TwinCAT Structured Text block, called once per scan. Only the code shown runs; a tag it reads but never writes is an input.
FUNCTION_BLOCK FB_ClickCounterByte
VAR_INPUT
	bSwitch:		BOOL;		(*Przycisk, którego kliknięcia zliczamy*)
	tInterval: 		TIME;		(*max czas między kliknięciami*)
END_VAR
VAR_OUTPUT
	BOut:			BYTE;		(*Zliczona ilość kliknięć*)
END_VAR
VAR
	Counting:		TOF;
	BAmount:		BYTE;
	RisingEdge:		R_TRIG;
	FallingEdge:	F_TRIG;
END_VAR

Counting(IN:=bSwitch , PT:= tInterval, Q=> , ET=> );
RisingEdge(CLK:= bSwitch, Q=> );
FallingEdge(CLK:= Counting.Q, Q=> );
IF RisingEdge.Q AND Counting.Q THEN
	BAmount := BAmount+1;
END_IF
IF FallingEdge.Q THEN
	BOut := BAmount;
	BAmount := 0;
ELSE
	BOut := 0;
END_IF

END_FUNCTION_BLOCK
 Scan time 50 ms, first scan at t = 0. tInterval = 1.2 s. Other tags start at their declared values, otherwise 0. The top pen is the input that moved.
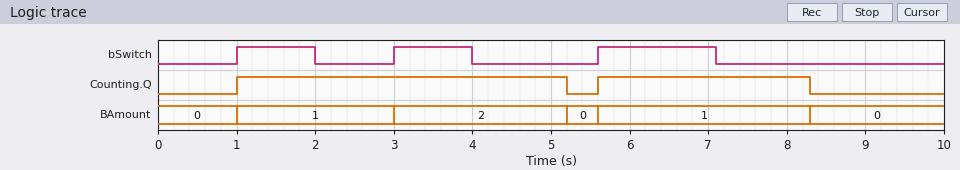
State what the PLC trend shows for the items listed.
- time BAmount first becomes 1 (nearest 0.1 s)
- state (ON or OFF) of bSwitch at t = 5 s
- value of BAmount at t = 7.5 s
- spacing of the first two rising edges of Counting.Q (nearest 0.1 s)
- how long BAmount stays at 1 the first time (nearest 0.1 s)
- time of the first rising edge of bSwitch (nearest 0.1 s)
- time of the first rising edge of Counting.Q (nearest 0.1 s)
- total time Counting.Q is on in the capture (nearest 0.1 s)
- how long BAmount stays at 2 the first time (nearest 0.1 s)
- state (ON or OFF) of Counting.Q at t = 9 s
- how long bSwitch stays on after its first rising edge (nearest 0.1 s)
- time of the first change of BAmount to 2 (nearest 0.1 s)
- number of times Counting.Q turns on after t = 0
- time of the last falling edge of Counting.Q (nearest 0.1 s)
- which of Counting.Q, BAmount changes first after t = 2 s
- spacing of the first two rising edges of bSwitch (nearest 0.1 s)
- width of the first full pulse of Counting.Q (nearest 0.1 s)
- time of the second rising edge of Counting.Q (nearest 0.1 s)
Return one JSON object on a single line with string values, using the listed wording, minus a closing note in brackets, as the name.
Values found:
{"time BAmount first becomes 1": "1.0 s", "state (ON or OFF) of bSwitch at t = 5 s": "OFF", "value of BAmount at t = 7.5 s": "1", "spacing of the first two rising edges of Counting.Q": "4.6 s", "how long BAmount stays at 1 the first time": "2.0 s", "time of the first rising edge of bSwitch": "1.0 s", "time of the first rising edge of Counting.Q": "1.0 s", "total time Counting.Q is on in the capture": "6.9 s", "how long BAmount stays at 2 the first time": "2.2 s", "state (ON or OFF) of Counting.Q at t = 9 s": "OFF", "how long bSwitch stays on after its first rising edge": "1.0 s", "time of the first change of BAmount to 2": "3.0 s", "number of times Counting.Q turns on after t = 0": "2", "time of the last falling edge of Counting.Q": "8.3 s", "which of Counting.Q, BAmount changes first after t = 2 s": "BAmount", "spacing of the first two rising edges of bSwitch": "2.0 s", "width of the first full pulse of Counting.Q": "4.2 s", "time of the second rising edge of Counting.Q": "5.6 s"}
